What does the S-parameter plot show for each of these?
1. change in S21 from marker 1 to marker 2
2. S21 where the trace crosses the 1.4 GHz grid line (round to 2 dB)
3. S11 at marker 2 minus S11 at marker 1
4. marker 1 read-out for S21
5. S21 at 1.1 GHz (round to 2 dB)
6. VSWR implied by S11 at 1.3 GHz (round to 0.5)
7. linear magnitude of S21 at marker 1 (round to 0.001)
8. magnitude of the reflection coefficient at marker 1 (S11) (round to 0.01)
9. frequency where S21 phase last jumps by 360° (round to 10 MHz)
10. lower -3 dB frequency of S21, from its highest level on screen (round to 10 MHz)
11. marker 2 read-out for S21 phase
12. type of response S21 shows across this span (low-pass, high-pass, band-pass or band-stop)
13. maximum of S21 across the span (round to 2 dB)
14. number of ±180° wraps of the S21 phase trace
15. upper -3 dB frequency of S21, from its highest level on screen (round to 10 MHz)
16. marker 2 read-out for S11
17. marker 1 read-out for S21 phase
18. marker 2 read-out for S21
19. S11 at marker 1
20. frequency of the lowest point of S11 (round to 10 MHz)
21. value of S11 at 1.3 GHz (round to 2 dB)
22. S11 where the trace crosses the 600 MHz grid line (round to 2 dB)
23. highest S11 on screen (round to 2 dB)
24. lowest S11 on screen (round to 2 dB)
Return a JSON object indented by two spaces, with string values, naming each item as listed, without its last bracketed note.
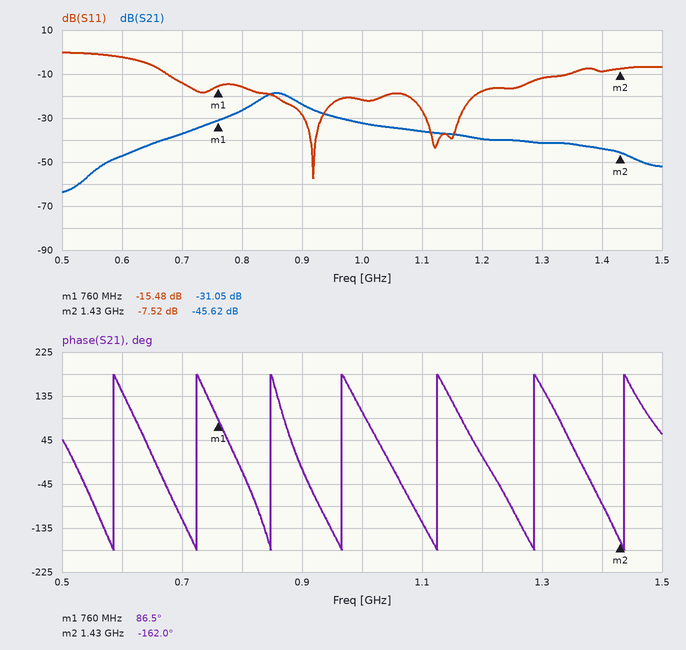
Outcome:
{
  "change in S21 from marker 1 to marker 2": "-14.57 dB",
  "S21 where the trace crosses the 1.4 GHz grid line": "-44 dB",
  "S11 at marker 2 minus S11 at marker 1": "7.96 dB",
  "marker 1 read-out for S21": "-31.05 dB",
  "S21 at 1.1 GHz": "-36 dB",
  "VSWR implied by S11 at 1.3 GHz": "1.5",
  "linear magnitude of S21 at marker 1": "0.028",
  "magnitude of the reflection coefficient at marker 1 (S11)": "0.17",
  "frequency where S21 phase last jumps by 360°": "1.44 GHz",
  "lower -3 dB frequency of S21, from its highest level on screen": "830 MHz",
  "marker 2 read-out for S21 phase": "-162.0°",
  "type of response S21 shows across this span": "band-pass",
  "maximum of S21 across the span": "-18 dB",
  "number of ±180° wraps of the S21 phase trace": "7",
  "upper -3 dB frequency of S21, from its highest level on screen": "890 MHz",
  "marker 2 read-out for S11": "-7.52 dB",
  "marker 1 read-out for S21 phase": "86.5°",
  "marker 2 read-out for S21": "-45.62 dB",
  "S11 at marker 1": "-15.48 dB",
  "frequency of the lowest point of S11": "920 MHz",
  "value of S11 at 1.3 GHz": "-12 dB",
  "S11 where the trace crosses the 600 MHz grid line": "-2 dB",
  "highest S11 on screen": "0 dB",
  "lowest S11 on screen": "-58 dB"
}
